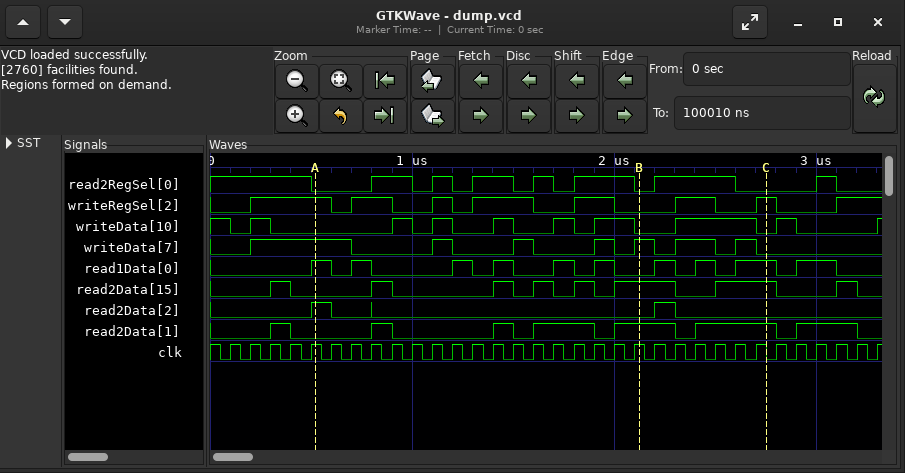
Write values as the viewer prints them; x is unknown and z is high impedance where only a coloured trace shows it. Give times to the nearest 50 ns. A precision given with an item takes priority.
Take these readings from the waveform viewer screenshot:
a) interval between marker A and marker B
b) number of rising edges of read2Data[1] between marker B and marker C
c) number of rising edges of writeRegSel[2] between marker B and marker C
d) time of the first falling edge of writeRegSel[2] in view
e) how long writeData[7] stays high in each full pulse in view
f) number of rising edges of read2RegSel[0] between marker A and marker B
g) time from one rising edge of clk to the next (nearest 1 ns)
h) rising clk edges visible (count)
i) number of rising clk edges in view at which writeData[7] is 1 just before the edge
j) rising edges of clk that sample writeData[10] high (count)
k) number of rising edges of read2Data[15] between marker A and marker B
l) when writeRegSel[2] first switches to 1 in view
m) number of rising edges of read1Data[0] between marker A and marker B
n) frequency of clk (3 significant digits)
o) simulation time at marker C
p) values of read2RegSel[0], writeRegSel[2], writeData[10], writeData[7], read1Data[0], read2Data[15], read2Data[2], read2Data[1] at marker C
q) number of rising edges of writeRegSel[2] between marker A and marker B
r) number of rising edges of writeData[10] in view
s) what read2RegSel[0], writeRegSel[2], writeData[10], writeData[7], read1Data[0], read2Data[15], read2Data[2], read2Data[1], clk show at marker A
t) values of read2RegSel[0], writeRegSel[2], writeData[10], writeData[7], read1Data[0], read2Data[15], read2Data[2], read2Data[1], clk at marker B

1600 ns
1
2
600 ns
500 ns, 100 ns, 100 ns, 100 ns, 100 ns, 200 ns, 100 ns
5
100 ns
33
12
13
5
200 ns
5
10.0 MHz
2750 ns
read2RegSel[0]=0, writeRegSel[2]=1, writeData[10]=0, writeData[7]=0, read1Data[0]=1, read2Data[15]=1, read2Data[2]=0, read2Data[1]=1
4
9
read2RegSel[0]=0, writeRegSel[2]=1, writeData[10]=0, writeData[7]=1, read1Data[0]=1, read2Data[15]=0, read2Data[2]=1, read2Data[1]=0, clk=1
read2RegSel[0]=0, writeRegSel[2]=0, writeData[10]=0, writeData[7]=1, read1Data[0]=0, read2Data[15]=1, read2Data[2]=0, read2Data[1]=1, clk=1
